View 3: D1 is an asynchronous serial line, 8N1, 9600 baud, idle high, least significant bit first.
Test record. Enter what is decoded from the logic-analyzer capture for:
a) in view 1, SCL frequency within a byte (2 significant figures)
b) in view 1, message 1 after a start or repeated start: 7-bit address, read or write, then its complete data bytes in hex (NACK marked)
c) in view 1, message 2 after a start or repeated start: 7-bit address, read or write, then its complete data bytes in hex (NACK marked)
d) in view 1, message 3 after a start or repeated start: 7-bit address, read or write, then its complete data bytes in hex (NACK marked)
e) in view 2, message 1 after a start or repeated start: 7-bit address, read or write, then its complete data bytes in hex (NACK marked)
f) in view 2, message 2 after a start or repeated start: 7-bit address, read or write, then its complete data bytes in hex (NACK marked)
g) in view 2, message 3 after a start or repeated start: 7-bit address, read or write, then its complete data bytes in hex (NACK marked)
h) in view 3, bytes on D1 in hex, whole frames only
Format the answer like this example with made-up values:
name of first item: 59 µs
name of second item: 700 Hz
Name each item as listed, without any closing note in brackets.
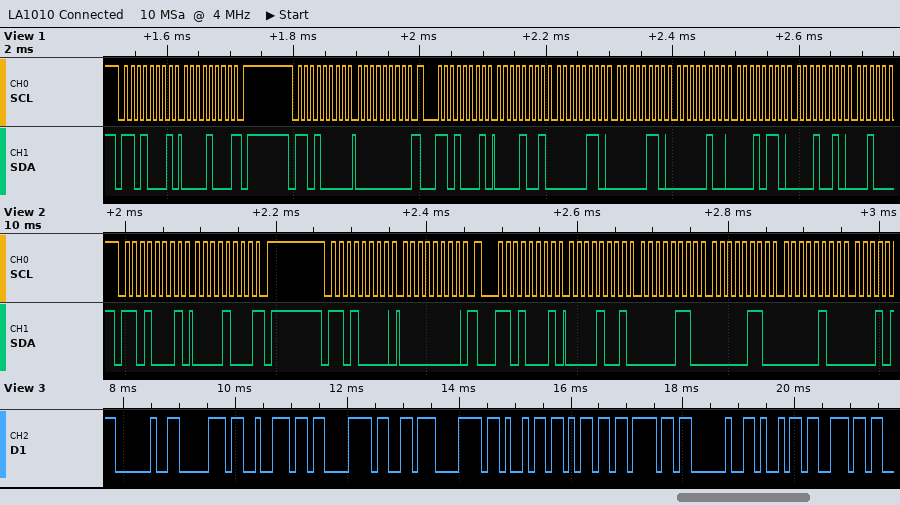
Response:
in view 1, SCL frequency within a byte: 100 kHz
in view 1, message 1 after a start or repeated start: 7-bit address, read or write, then its complete data bytes in hex: 0x68 read: 08 NACK
in view 1, message 2 after a start or repeated start: 7-bit address, read or write, then its complete data bytes in hex: 0x68 write: 00
in view 1, message 3 after a start or repeated start: 7-bit address, read or write, then its complete data bytes in hex: 0x68 read: 09 06 06 04 16 12
in view 2, message 1 after a start or repeated start: 7-bit address, read or write, then its complete data bytes in hex: 0x68 read: 08 NACK
in view 2, message 2 after a start or repeated start: 7-bit address, read or write, then its complete data bytes in hex: 0x68 write: 00
in view 2, message 3 after a start or repeated start: 7-bit address, read or write, then its complete data bytes in hex: 0x68 read: 09 06 06 04
in view 3, bytes on D1 in hex, whole frames only: 0x20 0x70 0x72 0xC3 0xB3 0x78 0x69 0x6D 0x6F 0x20 0x69 0x6E
